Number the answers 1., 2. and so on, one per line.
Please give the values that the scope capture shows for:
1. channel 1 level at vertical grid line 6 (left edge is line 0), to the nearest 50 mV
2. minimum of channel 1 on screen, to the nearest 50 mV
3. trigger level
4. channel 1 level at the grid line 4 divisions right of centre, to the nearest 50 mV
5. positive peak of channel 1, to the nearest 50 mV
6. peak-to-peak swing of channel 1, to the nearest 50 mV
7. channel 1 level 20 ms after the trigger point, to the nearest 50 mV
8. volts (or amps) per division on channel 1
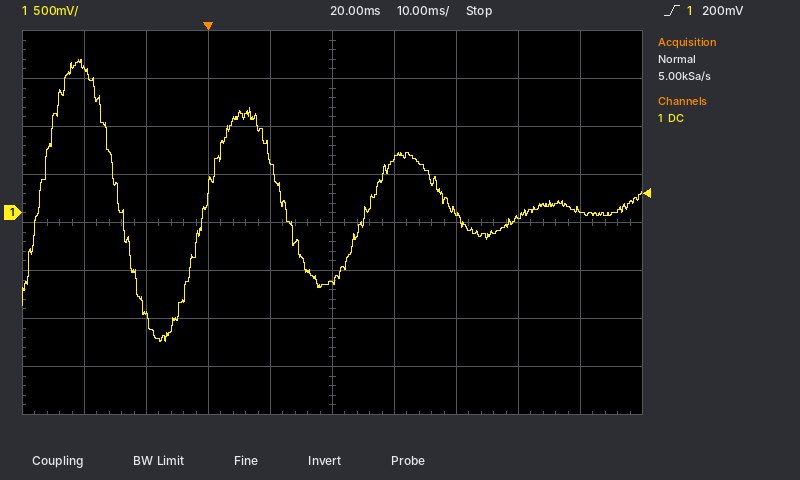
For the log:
1. 550 mV
2. -1.35 V
3. 200 mV
4. 50 mV
5. 1.60 V
6. 2.95 V
7. -700 mV
8. 500 mV
